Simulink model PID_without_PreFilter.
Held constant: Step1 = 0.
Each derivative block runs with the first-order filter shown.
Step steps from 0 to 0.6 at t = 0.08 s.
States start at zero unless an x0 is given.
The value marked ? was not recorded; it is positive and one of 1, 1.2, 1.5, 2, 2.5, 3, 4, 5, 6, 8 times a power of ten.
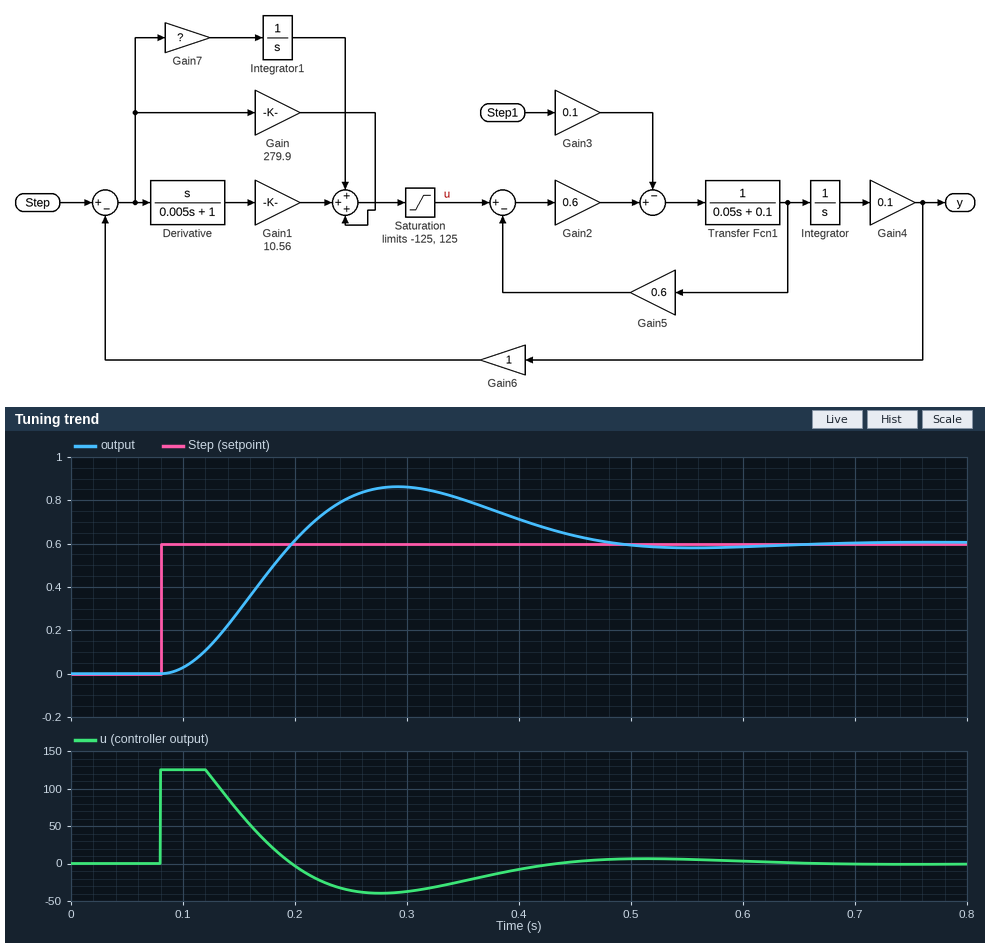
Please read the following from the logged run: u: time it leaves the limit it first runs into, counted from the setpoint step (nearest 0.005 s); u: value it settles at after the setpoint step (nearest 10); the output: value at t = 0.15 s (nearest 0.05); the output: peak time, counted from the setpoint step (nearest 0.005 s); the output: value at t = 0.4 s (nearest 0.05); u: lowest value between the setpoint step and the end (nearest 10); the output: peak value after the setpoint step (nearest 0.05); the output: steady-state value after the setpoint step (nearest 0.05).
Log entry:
0.040 s
0
0.30
0.210 s
0.70
-40
0.85
0.60
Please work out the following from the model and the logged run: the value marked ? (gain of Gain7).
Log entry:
1500
